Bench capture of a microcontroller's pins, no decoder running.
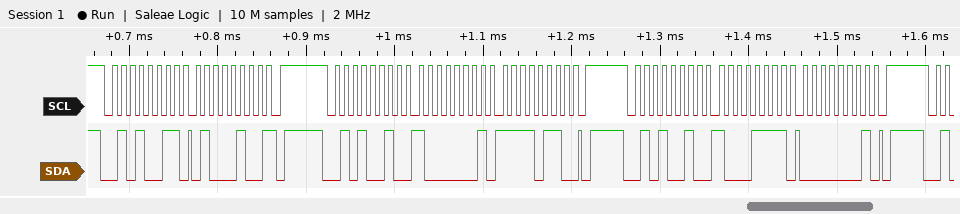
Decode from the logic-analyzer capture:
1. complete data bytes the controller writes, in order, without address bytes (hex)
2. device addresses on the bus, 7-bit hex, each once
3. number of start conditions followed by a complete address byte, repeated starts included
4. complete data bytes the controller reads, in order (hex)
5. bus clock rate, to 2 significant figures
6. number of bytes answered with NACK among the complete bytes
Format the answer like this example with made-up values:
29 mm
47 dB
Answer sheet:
81 F6 8F 01
0x29
3
44
100 kHz
1
